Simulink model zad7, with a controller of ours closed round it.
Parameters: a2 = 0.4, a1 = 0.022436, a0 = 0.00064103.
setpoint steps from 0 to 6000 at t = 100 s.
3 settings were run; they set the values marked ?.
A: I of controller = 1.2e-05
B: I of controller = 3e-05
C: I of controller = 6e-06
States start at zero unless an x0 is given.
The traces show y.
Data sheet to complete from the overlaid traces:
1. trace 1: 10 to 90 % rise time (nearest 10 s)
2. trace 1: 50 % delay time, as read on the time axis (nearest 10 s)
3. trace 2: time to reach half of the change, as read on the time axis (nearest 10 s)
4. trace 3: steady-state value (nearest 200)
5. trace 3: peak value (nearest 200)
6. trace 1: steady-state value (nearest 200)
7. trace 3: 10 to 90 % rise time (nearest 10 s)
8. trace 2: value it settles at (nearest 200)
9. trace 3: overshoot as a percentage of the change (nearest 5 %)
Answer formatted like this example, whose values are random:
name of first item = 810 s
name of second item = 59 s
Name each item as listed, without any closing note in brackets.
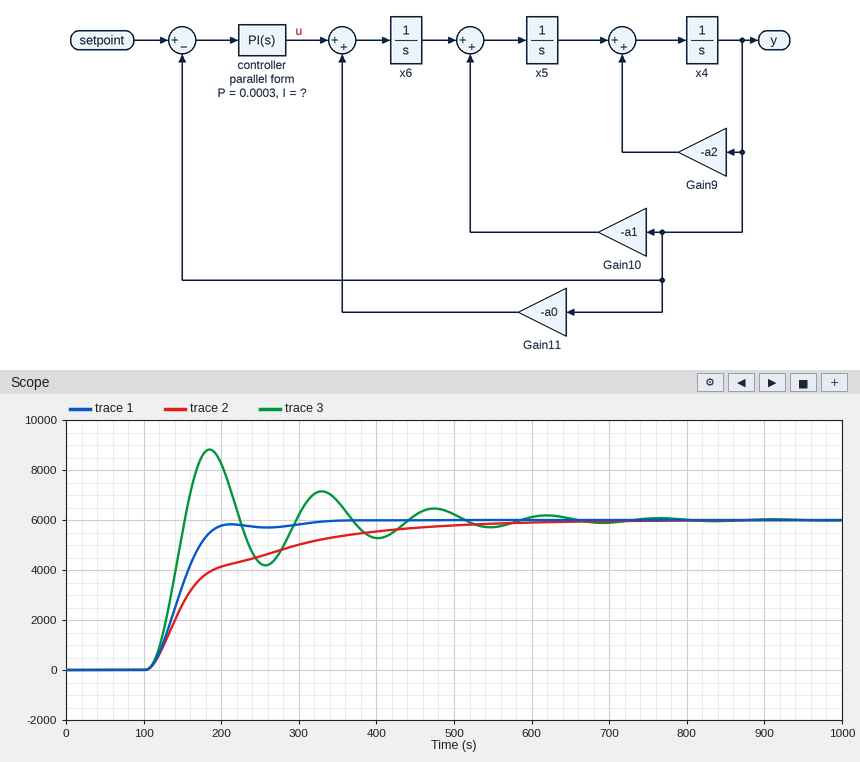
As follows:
trace 1: 10 to 90 % rise time = 60 s
trace 1: 50 % delay time, as read on the time axis = 150 s
trace 2: time to reach half of the change, as read on the time axis = 160 s
trace 3: steady-state value = 6000
trace 3: peak value = 8800
trace 1: steady-state value = 6000
trace 3: 10 to 90 % rise time = 30 s
trace 2: value it settles at = 6000
trace 3: overshoot as a percentage of the change = 45 %
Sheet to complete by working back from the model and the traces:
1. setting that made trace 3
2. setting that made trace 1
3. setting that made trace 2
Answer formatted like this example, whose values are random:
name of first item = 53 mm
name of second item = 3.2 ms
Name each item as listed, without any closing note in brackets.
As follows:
setting that made trace 3 = B
setting that made trace 1 = A
setting that made trace 2 = C
